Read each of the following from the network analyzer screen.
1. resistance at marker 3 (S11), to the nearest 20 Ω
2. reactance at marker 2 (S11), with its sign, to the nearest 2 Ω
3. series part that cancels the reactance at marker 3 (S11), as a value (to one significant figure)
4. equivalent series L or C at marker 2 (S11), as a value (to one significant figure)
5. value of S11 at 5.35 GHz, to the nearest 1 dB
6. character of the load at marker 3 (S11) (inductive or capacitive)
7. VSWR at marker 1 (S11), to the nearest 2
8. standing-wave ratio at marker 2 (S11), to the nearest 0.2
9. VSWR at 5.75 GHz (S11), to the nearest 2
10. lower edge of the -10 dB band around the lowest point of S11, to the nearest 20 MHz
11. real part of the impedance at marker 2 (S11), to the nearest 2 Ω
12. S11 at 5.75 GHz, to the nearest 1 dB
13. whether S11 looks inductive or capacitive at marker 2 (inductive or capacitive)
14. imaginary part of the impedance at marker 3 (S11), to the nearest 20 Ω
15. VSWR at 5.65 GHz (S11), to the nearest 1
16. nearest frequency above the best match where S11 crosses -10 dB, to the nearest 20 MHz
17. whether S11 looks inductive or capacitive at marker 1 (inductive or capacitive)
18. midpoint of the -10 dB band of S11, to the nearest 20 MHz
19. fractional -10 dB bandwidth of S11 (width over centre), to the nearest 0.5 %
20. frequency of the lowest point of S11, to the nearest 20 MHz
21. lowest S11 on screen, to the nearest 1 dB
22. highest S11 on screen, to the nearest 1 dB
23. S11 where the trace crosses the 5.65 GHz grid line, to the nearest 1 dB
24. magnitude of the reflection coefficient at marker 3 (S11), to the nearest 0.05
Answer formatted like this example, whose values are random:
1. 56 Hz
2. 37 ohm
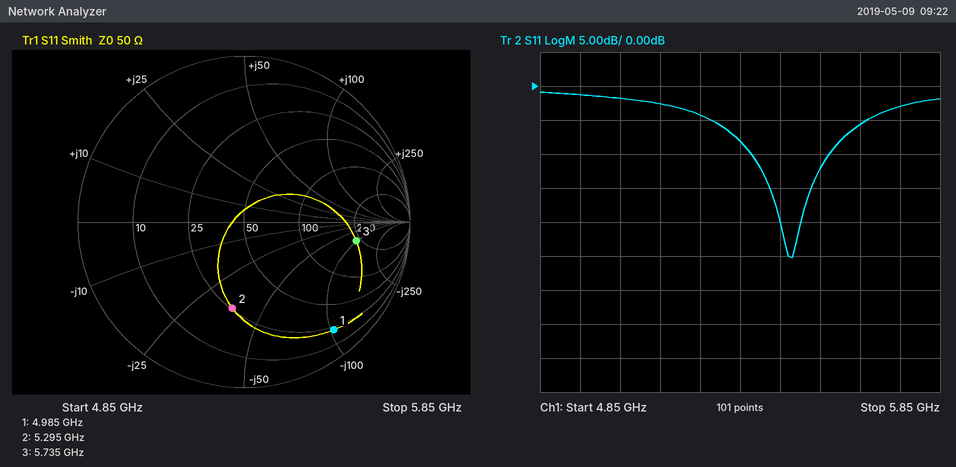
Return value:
1. 220 Ω
2. -36 Ω
3. 3 nH
4. 800 fF
5. -8 dB
6. capacitive
7. 12
8. 3.2
9. 6
10. 5.38 GHz
11. 26 Ω
12. -3 dB
13. capacitive
14. -100 Ω
15. 3
16. 5.58 GHz
17. capacitive
18. 5.48 GHz
19. 3.5 %
20. 5.48 GHz
21. -25 dB
22. -1 dB
23. -6 dB
24. 0.70
